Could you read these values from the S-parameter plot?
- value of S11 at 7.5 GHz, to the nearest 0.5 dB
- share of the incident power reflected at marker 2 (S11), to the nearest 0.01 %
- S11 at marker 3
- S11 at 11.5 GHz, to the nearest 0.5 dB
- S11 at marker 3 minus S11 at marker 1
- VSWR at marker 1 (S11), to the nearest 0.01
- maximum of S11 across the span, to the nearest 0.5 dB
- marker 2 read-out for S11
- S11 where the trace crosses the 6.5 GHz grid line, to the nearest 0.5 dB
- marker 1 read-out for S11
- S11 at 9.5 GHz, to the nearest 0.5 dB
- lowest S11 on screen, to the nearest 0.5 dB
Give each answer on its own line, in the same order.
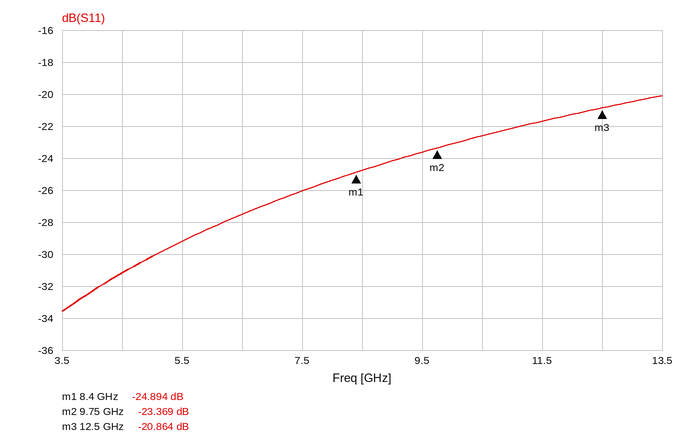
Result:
-26.0 dB
0.46 %
-20.864 dB
-21.5 dB
4.030 dB
1.12
-20.0 dB
-23.369 dB
-27.5 dB
-24.894 dB
-23.5 dB
-33.5 dB
